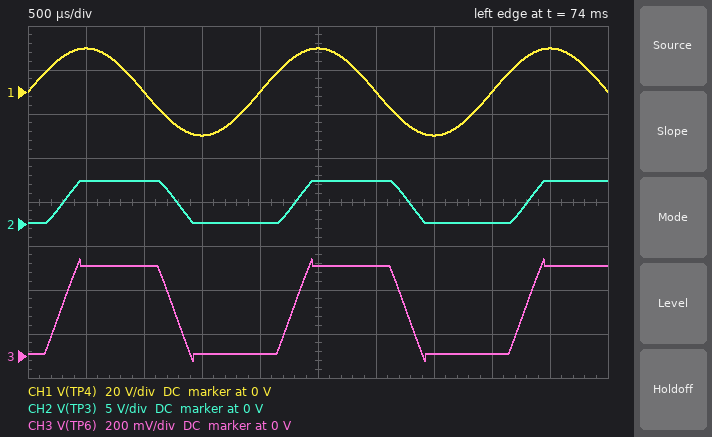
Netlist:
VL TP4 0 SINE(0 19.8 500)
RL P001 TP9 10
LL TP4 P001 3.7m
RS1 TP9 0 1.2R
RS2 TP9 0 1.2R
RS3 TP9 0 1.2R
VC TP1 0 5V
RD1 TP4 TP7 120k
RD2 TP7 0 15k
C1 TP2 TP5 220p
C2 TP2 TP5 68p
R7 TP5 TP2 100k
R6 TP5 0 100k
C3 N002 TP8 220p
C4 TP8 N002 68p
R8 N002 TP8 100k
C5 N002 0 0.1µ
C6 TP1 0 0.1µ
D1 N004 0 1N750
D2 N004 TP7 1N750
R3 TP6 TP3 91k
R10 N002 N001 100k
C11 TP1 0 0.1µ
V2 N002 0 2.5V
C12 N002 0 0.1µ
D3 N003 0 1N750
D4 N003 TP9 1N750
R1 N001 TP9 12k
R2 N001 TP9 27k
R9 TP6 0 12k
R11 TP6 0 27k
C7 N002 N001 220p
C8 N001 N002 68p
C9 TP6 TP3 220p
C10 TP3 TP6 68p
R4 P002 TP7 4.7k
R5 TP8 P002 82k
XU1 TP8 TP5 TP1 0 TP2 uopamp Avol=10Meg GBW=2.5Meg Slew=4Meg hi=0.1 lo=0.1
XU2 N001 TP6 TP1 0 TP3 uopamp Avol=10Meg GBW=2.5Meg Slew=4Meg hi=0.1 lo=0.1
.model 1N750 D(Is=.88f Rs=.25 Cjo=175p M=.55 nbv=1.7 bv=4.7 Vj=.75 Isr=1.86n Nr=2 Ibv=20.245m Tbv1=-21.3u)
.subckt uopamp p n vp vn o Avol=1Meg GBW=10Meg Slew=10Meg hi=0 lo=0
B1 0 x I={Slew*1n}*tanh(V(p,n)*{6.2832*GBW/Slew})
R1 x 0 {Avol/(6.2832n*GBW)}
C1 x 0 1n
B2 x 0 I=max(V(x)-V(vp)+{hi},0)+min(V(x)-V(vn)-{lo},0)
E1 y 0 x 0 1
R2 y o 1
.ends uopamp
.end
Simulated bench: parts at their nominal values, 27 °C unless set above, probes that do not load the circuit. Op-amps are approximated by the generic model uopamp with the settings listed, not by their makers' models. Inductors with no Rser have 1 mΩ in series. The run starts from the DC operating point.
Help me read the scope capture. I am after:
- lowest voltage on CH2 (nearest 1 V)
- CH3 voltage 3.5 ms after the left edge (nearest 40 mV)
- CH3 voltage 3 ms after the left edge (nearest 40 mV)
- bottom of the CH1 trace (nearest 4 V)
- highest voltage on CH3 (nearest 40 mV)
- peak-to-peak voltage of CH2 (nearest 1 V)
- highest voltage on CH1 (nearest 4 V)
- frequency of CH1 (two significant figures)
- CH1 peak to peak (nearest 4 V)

0 V
0 V
400 mV
-20 V
440 mV
5 V
20 V
500 Hz
40 V
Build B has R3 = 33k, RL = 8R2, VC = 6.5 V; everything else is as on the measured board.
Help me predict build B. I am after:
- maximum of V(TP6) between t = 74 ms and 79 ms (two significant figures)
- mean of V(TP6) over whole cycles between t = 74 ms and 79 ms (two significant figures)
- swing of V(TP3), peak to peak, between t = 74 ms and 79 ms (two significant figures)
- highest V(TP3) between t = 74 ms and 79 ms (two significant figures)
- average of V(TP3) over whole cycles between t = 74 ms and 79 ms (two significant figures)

700 mV
280 mV
3.4 V
3.5 V
1.4 V
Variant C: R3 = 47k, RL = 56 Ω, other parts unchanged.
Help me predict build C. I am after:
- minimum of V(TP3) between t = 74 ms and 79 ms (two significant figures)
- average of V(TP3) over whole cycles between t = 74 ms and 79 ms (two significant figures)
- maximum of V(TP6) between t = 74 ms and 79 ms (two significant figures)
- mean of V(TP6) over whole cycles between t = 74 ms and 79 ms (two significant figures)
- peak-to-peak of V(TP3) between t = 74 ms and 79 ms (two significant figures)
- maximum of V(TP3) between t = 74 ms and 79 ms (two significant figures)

430 mV
1.3 V
320 mV
190 mV
1.7 V
2.1 V
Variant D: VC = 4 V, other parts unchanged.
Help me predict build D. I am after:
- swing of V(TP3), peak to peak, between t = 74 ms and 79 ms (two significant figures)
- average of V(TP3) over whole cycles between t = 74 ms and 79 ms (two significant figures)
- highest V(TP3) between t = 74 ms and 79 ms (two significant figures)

3.8 V
2.1 V
3.9 V
